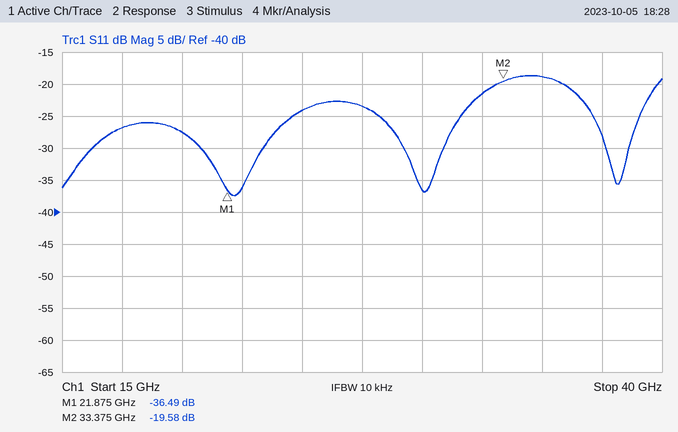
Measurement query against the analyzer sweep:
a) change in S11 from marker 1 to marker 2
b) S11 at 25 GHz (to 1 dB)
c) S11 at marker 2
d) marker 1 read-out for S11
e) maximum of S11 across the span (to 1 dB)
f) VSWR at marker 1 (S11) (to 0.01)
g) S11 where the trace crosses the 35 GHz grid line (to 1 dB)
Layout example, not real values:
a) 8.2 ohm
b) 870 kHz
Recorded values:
a) 16.91 dB
b) -24 dB
c) -19.58 dB
d) -36.49 dB
e) -19 dB
f) 1.03
g) -19 dB
